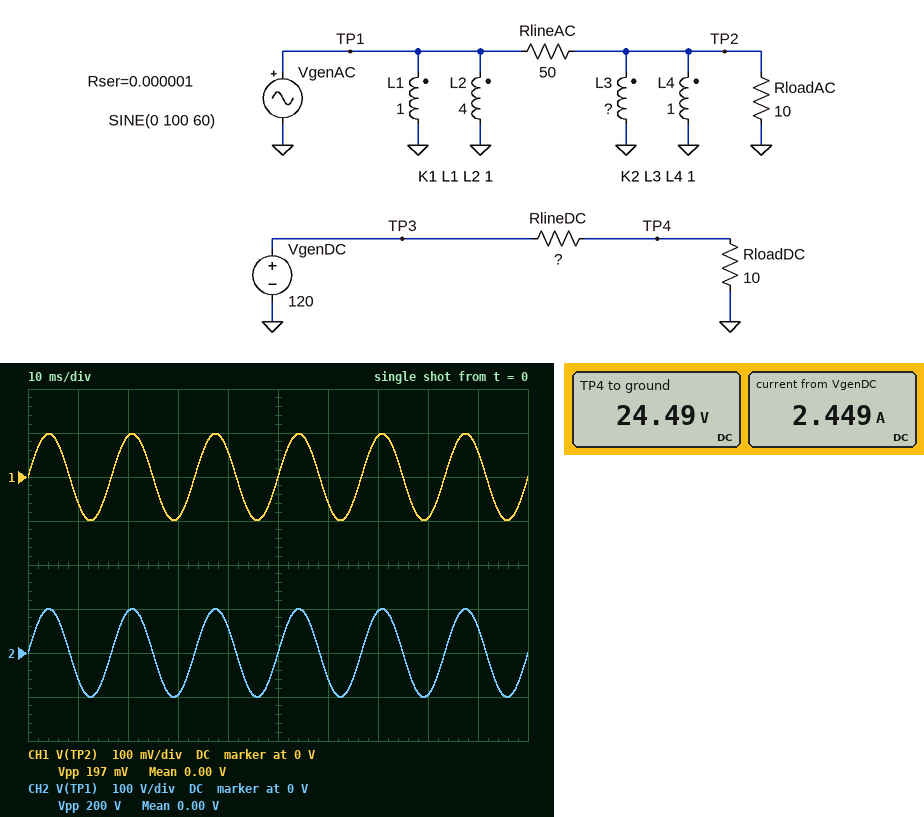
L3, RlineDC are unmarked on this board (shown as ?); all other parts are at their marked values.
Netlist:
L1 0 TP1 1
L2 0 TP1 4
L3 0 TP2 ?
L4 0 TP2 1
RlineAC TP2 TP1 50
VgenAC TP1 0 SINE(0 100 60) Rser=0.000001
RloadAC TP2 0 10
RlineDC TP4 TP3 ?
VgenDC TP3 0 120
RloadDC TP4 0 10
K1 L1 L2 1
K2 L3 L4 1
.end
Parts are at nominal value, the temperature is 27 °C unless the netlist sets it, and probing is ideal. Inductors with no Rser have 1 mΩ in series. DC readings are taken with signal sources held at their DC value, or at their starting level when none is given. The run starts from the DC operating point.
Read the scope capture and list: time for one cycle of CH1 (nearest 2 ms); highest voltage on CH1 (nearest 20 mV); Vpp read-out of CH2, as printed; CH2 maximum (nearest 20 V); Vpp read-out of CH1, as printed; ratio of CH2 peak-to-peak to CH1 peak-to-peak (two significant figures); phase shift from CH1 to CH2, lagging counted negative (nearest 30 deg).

16 ms
100 mV
200 V
100 V
197 mV
1000
0 deg
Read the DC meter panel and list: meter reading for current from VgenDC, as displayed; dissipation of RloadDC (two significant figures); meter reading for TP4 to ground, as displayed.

2.449 A
60 W
24.49 V
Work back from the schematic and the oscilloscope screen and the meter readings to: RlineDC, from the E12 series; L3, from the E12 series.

39 Ω
1.5 H
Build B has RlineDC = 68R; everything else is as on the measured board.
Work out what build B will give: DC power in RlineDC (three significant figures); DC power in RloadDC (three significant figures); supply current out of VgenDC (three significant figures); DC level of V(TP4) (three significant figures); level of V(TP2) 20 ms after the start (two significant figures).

161 W
23.7 W
1.54 A
15.4 V
94 mV
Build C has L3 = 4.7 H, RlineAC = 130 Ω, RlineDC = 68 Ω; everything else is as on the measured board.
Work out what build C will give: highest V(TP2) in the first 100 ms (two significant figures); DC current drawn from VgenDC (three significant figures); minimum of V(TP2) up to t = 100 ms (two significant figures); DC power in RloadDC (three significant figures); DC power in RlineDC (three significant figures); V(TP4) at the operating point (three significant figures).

3.2 mV
1.54 A
-3.2 mV
23.7 W
161 W
15.4 V
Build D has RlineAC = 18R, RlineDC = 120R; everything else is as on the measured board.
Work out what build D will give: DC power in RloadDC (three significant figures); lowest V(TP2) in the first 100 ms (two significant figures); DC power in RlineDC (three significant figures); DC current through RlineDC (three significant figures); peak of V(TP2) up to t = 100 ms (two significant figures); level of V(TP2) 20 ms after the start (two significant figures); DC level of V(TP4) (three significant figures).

8.52 W
-270 mV
102 W
923 mA
270 mV
260 mV
9.23 V
